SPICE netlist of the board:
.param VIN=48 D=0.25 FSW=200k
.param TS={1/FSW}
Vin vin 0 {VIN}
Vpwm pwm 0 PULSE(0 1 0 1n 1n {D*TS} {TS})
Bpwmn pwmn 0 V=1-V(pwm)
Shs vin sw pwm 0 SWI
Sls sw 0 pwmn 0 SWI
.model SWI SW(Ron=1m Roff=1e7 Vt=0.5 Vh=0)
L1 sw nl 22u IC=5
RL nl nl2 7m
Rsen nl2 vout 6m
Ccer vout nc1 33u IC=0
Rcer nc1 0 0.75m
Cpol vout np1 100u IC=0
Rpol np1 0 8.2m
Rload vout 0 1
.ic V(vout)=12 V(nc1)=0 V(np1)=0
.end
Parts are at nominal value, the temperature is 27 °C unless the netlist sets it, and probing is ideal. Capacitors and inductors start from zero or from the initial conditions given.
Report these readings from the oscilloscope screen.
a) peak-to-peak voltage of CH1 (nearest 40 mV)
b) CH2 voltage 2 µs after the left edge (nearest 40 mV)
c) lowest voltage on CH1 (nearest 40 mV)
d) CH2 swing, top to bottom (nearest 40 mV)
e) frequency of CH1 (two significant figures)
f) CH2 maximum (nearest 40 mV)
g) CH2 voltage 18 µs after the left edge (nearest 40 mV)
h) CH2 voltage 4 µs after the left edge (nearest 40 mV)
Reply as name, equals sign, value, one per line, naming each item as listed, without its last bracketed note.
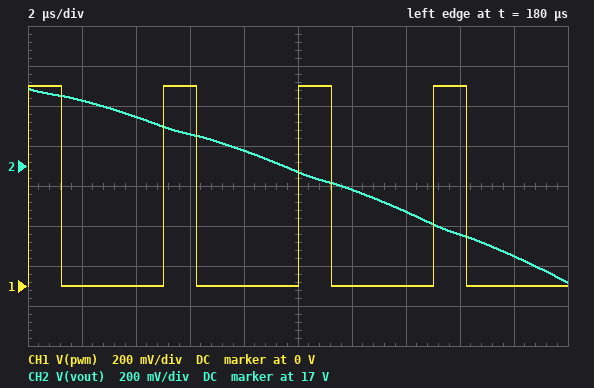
peak-to-peak voltage of CH1 = 1.00 V
CH2 voltage 2 µs after the left edge = 17.32 V
lowest voltage on CH1 = 0 V
CH2 swing, top to bottom = 960 mV
frequency of CH1 = 200 kHz
CH2 maximum = 17.40 V
CH2 voltage 18 µs after the left edge = 16.56 V
CH2 voltage 4 µs after the left edge = 17.24 V
